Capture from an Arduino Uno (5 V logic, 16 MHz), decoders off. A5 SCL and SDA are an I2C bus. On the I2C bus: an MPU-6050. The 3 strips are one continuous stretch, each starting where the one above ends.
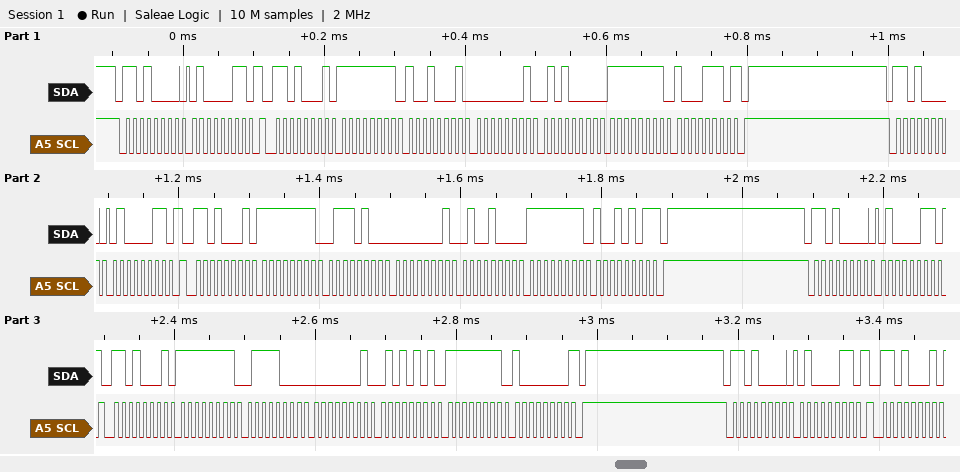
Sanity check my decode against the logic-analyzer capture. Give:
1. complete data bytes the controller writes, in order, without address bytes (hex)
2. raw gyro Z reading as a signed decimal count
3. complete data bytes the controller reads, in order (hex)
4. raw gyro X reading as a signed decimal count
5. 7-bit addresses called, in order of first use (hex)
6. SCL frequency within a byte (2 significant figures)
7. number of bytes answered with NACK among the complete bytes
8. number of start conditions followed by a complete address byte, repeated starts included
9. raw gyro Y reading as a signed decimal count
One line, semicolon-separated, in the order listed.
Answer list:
43 43 43 43; -114; FF 91 01 50 FF 8E FF 74 01 48 FF 95 FF 78 01 55 FF 80; -111; 0x68; 100 kHz; 3; 8; 336
